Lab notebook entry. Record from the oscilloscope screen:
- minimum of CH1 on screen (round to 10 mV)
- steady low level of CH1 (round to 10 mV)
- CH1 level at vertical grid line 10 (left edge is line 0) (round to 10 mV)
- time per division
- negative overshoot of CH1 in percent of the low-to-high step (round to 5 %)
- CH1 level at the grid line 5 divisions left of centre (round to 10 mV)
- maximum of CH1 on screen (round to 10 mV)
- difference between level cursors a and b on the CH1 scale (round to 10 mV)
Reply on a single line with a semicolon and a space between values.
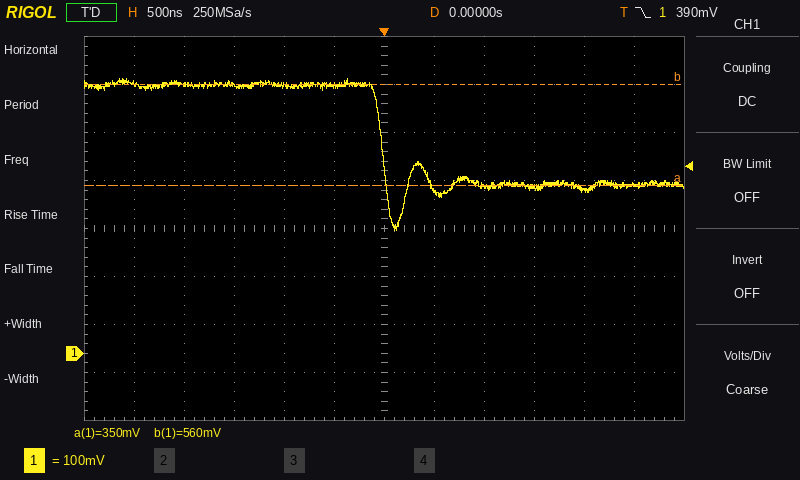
260 mV; 350 mV; 340 mV; 500 ns; 45 %; 560 mV; 570 mV; 210 mV
